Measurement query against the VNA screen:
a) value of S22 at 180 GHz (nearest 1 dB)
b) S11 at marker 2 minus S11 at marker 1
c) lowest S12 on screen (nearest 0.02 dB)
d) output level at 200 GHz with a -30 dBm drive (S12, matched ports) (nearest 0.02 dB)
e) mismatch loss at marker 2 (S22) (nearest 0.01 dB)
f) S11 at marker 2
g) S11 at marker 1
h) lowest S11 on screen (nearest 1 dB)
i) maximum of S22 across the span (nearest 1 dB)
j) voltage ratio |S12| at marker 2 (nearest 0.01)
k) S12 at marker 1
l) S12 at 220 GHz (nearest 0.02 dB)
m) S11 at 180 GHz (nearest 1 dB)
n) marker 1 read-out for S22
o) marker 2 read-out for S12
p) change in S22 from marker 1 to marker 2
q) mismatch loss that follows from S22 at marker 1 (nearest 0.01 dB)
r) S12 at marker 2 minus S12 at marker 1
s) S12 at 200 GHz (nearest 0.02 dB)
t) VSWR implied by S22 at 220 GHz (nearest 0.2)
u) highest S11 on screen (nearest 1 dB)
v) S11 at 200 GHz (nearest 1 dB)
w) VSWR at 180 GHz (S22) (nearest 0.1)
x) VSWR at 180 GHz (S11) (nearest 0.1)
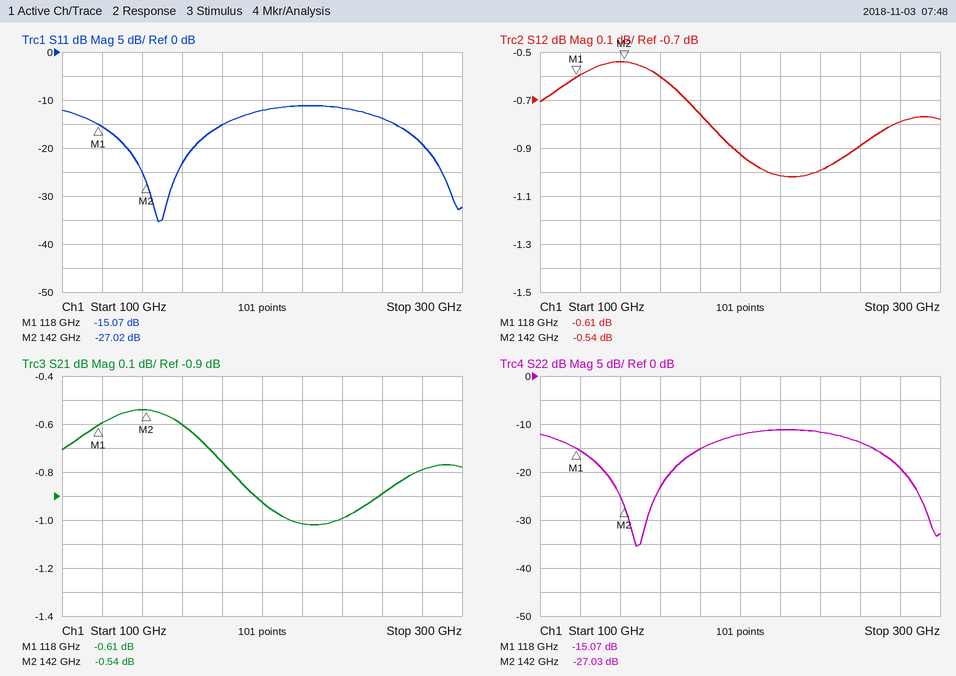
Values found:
-15 dB
-11.95 dB
-1.02 dB
-30.92 dBm
0.01 dB
-27.02 dB
-15.07 dB
-35 dB
-11 dB
0.94
-0.61 dB
-1.02 dB
-15 dB
-15.07 dB
-0.54 dB
-11.96 dB
0.14 dB
0.07 dB
-0.92 dB
1.8
-11 dB
-12 dB
1.4
1.4
